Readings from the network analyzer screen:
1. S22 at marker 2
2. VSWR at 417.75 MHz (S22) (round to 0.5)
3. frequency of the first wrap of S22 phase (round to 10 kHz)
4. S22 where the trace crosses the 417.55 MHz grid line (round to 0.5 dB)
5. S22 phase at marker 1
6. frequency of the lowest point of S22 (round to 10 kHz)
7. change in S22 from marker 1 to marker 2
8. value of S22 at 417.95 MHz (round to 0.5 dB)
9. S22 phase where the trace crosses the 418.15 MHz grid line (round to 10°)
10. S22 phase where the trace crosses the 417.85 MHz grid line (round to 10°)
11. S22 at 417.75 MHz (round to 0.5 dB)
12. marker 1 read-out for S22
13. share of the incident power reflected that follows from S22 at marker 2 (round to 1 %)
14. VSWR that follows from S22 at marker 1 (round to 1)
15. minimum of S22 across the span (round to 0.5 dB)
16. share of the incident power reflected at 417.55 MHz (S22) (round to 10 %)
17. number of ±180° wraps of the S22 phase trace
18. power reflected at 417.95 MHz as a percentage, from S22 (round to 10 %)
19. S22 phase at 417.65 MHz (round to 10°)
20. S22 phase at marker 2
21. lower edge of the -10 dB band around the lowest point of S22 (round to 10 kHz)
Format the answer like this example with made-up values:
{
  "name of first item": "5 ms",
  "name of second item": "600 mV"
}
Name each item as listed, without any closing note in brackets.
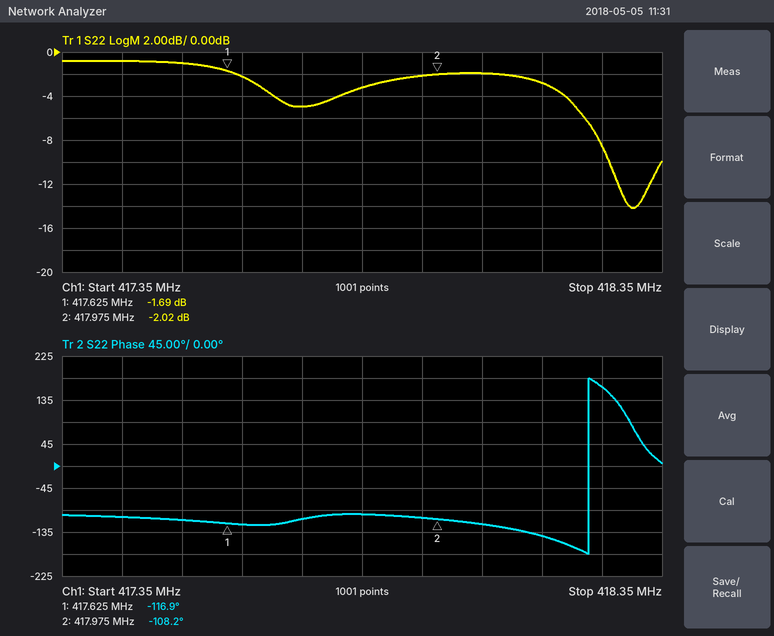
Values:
{
  "S22 at marker 2": "-2.02 dB",
  "VSWR at 417.75 MHz (S22)": "3.5",
  "frequency of the first wrap of S22 phase": "418.23 MHz",
  "S22 where the trace crosses the 417.55 MHz grid line": "-1.0 dB",
  "S22 phase at marker 1": "-116.9°",
  "frequency of the lowest point of S22": "418.30 MHz",
  "change in S22 from marker 1 to marker 2": "-0.33 dB",
  "value of S22 at 417.95 MHz": "-2.0 dB",
  "S22 phase where the trace crosses the 418.15 MHz grid line": "-140°",
  "S22 phase where the trace crosses the 417.85 MHz grid line": "-100°",
  "S22 at 417.75 MHz": "-5.0 dB",
  "marker 1 read-out for S22": "-1.69 dB",
  "share of the incident power reflected that follows from S22 at marker 2": "63 %",
  "VSWR that follows from S22 at marker 1": "10",
  "minimum of S22 across the span": "-14.0 dB",
  "share of the incident power reflected at 417.55 MHz (S22)": "80 %",
  "number of ±180° wraps of the S22 phase trace": "1",
  "power reflected at 417.95 MHz as a percentage, from S22": "60 %",
  "S22 phase at 417.65 MHz": "-120°",
  "S22 phase at marker 2": "-108.2°",
  "lower edge of the -10 dB band around the lowest point of S22": "418.26 MHz"
}
